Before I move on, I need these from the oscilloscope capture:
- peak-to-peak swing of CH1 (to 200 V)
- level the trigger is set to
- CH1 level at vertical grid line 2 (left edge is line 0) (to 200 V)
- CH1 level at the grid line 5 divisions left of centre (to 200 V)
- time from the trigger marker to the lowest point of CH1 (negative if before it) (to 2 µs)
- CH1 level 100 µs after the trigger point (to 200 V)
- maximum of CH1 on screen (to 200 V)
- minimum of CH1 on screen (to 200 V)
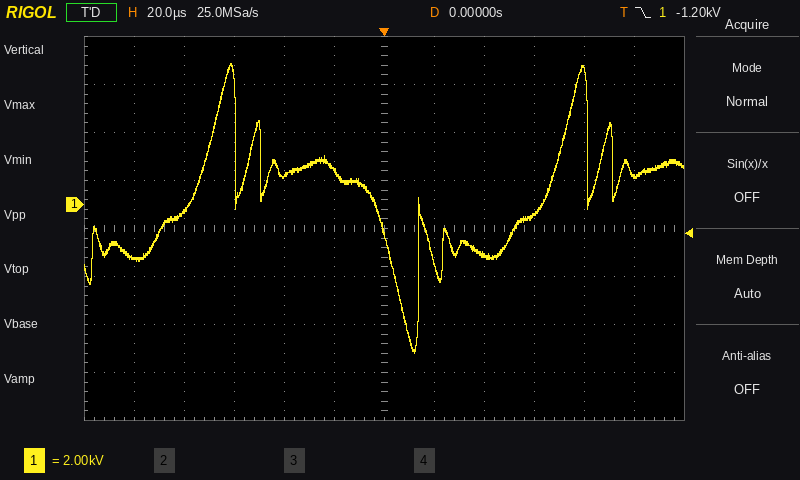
12.0 kV
-1.20 kV
-400 V
-2.2 kV
+12 µs
1.2 kV
5.8 kV
-6.2 kV
